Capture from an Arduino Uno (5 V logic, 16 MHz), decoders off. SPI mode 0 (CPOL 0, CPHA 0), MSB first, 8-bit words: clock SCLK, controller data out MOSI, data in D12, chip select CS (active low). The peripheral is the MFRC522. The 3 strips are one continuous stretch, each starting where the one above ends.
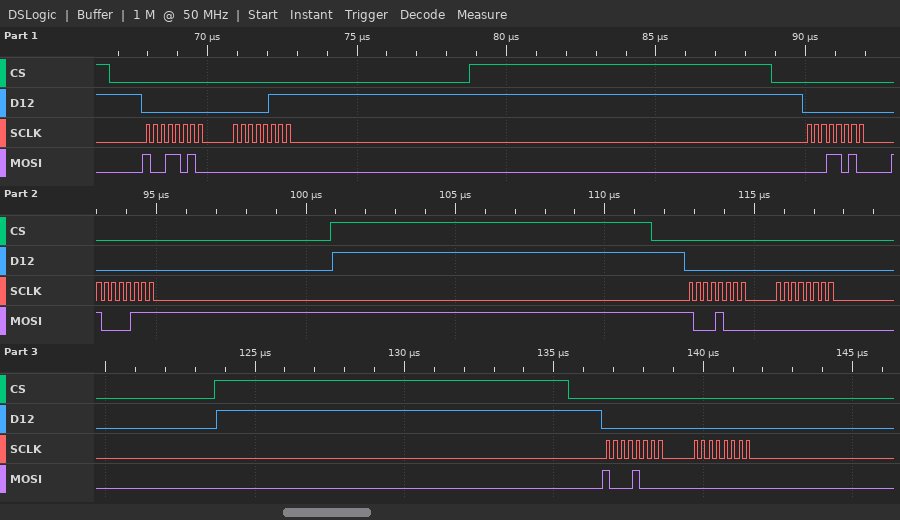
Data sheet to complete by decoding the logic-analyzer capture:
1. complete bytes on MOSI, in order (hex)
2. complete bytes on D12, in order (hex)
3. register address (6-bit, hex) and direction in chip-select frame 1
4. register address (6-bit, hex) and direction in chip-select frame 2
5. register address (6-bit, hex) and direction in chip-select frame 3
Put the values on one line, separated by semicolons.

0x9A 0x00 0x1A 0x87 0x88 0x00 0x88 0x00; 0x00 0x07 0x00 0x00 0x00 0x00 0x00 0x00; 0x0D read; 0x0D write; 0x04 read
